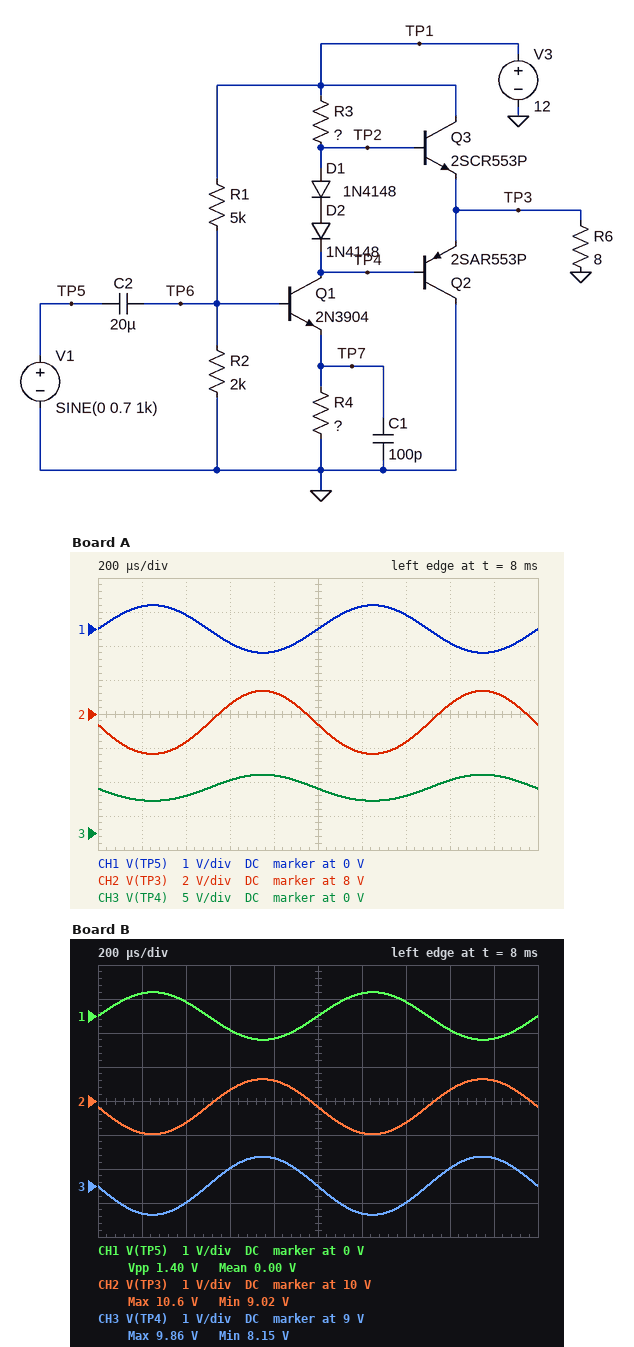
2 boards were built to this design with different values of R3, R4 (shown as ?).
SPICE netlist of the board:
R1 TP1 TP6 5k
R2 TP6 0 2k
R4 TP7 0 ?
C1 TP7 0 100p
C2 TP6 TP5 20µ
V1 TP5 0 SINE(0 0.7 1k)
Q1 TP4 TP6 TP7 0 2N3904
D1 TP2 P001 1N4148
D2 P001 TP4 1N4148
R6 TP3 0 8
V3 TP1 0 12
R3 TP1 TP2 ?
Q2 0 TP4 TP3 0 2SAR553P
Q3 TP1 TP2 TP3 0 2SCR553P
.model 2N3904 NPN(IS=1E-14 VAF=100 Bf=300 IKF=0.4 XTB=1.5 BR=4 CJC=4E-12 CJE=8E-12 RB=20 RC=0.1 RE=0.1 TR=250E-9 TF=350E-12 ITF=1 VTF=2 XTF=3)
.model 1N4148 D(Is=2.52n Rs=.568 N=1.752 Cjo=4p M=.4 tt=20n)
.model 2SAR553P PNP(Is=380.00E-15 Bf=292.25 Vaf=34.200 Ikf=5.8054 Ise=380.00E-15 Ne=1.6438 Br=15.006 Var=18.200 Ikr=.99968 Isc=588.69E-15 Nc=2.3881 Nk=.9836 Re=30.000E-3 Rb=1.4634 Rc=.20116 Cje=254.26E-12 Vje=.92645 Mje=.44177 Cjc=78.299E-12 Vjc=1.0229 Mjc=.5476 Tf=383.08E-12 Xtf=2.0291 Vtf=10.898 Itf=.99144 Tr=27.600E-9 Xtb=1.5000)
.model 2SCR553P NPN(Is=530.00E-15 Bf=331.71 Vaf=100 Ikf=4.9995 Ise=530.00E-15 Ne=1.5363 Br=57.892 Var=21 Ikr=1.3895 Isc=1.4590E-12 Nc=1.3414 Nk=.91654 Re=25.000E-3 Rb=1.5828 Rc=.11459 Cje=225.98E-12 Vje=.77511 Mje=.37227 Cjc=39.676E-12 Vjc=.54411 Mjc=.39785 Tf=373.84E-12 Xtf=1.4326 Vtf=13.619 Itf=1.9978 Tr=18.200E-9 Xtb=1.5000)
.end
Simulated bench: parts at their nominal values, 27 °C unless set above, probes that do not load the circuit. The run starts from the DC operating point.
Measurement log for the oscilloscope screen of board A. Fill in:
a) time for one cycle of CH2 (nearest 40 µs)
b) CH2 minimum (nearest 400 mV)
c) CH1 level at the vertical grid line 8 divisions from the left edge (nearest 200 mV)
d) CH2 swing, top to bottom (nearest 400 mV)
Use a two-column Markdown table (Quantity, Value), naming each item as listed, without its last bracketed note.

| Quantity | Value |
|---|---|
| time for one cycle of CH2 | 1.00 ms |
| CH2 minimum | 5.6 V |
| CH1 level at the vertical grid line 8 divisions from the left edge | -400 mV |
| CH2 swing, top to bottom | 3.6 V |
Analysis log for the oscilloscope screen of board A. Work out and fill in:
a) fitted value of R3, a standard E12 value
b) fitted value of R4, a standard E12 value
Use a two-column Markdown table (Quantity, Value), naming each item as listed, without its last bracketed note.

| Quantity | Value |
|---|---|
| fitted value of R3, a standard E12 value | 15 Ω |
| fitted value of R4, a standard E12 value | 6.8 Ω |
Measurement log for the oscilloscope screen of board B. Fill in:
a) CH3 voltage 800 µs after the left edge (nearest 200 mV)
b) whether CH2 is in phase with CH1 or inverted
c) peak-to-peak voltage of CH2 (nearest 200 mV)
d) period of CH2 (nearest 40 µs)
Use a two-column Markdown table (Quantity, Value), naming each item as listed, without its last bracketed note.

| Quantity | Value |
|---|---|
| CH3 voltage 800 µs after the left edge | 9.8 V |
| whether CH2 is in phase with CH1 or inverted | inverted |
| peak-to-peak voltage of CH2 | 1.6 V |
| period of CH2 | 1.00 ms |
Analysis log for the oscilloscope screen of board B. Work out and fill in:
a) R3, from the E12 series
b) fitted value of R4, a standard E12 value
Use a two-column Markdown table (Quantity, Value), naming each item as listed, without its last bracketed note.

| Quantity | Value |
|---|---|
| R3, from the E12 series | 3.9 Ω |
| fitted value of R4, a standard E12 value | 5.6 Ω |
